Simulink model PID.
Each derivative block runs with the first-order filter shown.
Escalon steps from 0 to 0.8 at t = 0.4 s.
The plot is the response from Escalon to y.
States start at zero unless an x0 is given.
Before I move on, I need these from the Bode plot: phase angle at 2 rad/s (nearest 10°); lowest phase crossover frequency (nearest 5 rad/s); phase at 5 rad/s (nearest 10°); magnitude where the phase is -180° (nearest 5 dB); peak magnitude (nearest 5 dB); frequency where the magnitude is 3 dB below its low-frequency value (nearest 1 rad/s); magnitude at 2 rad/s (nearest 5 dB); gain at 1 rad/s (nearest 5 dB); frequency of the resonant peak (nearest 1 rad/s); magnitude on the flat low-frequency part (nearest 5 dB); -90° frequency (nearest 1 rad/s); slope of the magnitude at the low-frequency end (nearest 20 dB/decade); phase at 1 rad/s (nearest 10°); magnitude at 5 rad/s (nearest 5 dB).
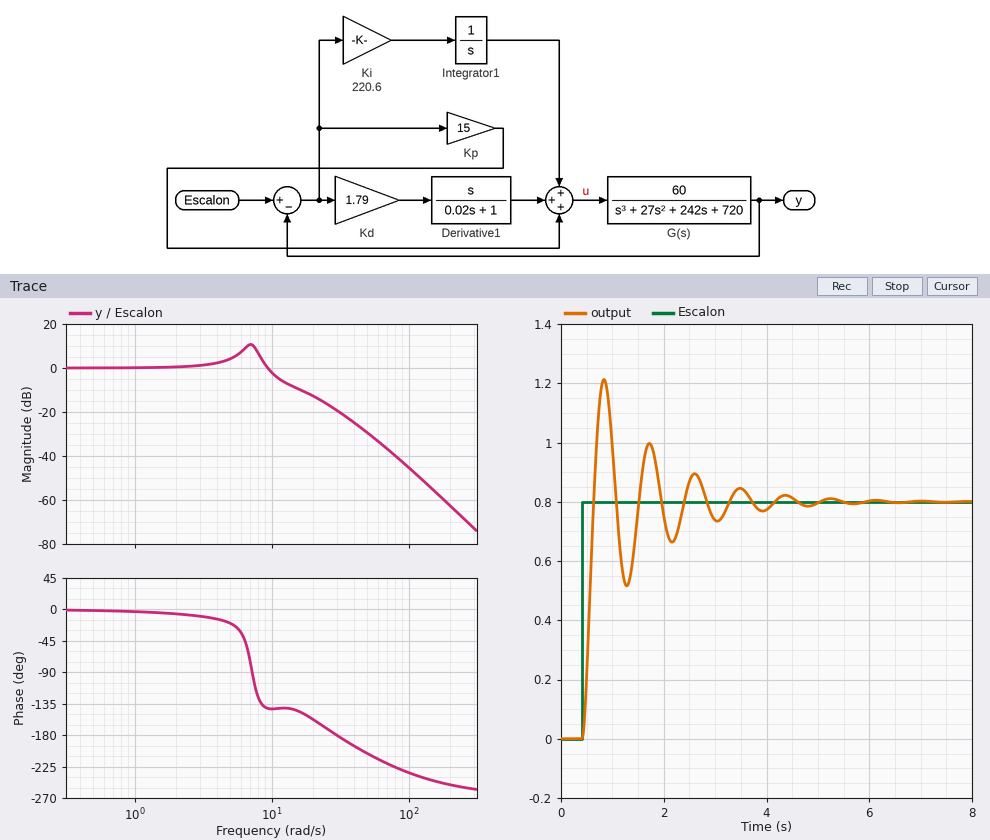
-10°
30 rad/s
-20°
-20 dB
10 dB
10 rad/s
0 dB
0 dB
7 rad/s
0 dB
7 rad/s
0 dB/decade
0°
5 dB
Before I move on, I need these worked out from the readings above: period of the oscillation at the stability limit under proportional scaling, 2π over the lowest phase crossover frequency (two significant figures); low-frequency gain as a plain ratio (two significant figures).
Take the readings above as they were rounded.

0.21 s
1.0
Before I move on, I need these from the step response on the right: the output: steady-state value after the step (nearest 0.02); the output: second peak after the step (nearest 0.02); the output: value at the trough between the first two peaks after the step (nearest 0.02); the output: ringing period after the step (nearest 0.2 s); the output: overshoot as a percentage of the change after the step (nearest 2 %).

0.80
1.00
0.52
0.8 s
52 %
